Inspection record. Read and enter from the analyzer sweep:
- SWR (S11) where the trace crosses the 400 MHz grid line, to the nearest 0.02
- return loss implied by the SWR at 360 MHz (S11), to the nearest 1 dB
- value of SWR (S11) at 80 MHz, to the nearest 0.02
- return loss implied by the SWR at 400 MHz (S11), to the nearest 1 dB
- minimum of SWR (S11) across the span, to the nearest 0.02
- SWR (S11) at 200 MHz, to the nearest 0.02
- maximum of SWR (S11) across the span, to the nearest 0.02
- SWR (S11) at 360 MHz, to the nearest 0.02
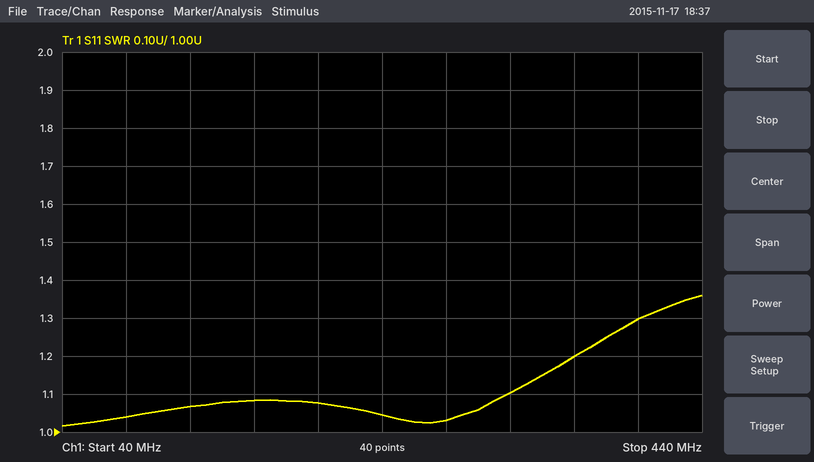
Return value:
1.30
21 dB
1.04
18 dB
1.02
1.08
1.36
1.20
